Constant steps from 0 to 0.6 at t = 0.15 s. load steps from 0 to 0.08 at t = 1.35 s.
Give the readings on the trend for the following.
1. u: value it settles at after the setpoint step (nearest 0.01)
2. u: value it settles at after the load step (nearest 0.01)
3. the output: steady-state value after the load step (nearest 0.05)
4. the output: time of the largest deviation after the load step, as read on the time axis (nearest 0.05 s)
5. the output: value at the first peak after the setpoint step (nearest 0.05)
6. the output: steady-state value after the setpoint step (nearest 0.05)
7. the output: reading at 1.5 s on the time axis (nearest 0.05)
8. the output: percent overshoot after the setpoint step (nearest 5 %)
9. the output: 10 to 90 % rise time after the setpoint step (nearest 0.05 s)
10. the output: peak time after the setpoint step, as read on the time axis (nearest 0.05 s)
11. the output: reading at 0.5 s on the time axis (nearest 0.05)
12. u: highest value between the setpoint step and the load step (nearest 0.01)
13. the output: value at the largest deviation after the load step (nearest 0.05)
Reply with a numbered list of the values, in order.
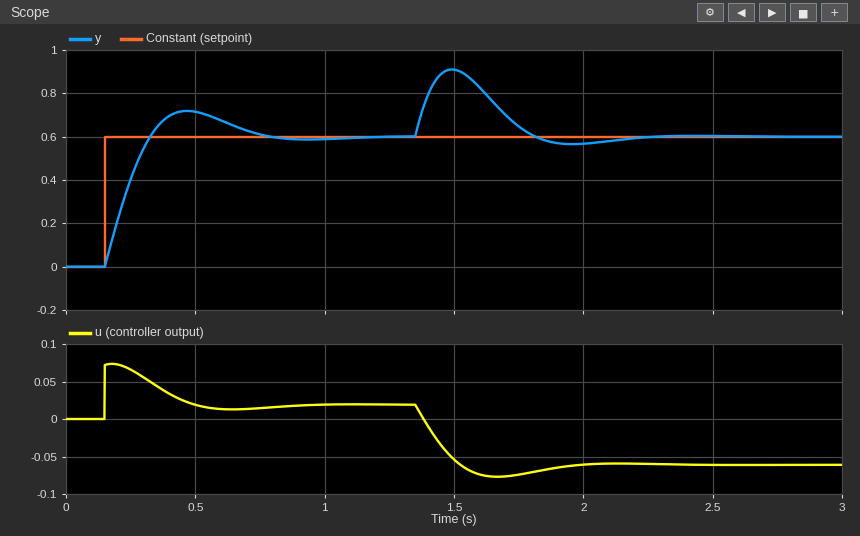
1. 0.02
2. -0.06
3. 0.60
4. 1.50 s
5. 0.70
6. 0.60
7. 0.90
8. 20 %
9. 0.15 s
10. 0.45 s
11. 0.70
12. 0.07
13. 0.90
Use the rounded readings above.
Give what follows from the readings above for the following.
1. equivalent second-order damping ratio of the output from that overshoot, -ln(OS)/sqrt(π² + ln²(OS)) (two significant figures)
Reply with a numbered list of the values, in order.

1. 0.46
